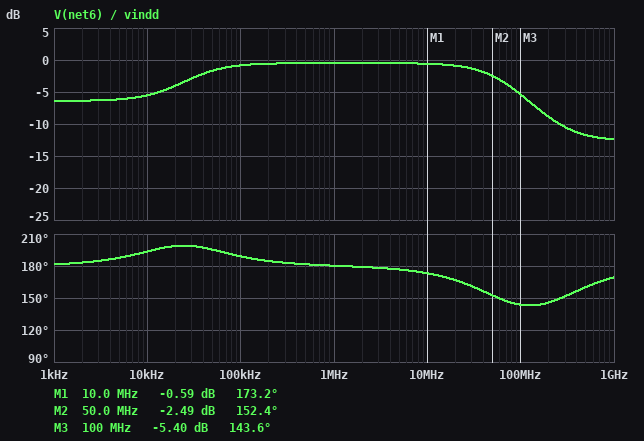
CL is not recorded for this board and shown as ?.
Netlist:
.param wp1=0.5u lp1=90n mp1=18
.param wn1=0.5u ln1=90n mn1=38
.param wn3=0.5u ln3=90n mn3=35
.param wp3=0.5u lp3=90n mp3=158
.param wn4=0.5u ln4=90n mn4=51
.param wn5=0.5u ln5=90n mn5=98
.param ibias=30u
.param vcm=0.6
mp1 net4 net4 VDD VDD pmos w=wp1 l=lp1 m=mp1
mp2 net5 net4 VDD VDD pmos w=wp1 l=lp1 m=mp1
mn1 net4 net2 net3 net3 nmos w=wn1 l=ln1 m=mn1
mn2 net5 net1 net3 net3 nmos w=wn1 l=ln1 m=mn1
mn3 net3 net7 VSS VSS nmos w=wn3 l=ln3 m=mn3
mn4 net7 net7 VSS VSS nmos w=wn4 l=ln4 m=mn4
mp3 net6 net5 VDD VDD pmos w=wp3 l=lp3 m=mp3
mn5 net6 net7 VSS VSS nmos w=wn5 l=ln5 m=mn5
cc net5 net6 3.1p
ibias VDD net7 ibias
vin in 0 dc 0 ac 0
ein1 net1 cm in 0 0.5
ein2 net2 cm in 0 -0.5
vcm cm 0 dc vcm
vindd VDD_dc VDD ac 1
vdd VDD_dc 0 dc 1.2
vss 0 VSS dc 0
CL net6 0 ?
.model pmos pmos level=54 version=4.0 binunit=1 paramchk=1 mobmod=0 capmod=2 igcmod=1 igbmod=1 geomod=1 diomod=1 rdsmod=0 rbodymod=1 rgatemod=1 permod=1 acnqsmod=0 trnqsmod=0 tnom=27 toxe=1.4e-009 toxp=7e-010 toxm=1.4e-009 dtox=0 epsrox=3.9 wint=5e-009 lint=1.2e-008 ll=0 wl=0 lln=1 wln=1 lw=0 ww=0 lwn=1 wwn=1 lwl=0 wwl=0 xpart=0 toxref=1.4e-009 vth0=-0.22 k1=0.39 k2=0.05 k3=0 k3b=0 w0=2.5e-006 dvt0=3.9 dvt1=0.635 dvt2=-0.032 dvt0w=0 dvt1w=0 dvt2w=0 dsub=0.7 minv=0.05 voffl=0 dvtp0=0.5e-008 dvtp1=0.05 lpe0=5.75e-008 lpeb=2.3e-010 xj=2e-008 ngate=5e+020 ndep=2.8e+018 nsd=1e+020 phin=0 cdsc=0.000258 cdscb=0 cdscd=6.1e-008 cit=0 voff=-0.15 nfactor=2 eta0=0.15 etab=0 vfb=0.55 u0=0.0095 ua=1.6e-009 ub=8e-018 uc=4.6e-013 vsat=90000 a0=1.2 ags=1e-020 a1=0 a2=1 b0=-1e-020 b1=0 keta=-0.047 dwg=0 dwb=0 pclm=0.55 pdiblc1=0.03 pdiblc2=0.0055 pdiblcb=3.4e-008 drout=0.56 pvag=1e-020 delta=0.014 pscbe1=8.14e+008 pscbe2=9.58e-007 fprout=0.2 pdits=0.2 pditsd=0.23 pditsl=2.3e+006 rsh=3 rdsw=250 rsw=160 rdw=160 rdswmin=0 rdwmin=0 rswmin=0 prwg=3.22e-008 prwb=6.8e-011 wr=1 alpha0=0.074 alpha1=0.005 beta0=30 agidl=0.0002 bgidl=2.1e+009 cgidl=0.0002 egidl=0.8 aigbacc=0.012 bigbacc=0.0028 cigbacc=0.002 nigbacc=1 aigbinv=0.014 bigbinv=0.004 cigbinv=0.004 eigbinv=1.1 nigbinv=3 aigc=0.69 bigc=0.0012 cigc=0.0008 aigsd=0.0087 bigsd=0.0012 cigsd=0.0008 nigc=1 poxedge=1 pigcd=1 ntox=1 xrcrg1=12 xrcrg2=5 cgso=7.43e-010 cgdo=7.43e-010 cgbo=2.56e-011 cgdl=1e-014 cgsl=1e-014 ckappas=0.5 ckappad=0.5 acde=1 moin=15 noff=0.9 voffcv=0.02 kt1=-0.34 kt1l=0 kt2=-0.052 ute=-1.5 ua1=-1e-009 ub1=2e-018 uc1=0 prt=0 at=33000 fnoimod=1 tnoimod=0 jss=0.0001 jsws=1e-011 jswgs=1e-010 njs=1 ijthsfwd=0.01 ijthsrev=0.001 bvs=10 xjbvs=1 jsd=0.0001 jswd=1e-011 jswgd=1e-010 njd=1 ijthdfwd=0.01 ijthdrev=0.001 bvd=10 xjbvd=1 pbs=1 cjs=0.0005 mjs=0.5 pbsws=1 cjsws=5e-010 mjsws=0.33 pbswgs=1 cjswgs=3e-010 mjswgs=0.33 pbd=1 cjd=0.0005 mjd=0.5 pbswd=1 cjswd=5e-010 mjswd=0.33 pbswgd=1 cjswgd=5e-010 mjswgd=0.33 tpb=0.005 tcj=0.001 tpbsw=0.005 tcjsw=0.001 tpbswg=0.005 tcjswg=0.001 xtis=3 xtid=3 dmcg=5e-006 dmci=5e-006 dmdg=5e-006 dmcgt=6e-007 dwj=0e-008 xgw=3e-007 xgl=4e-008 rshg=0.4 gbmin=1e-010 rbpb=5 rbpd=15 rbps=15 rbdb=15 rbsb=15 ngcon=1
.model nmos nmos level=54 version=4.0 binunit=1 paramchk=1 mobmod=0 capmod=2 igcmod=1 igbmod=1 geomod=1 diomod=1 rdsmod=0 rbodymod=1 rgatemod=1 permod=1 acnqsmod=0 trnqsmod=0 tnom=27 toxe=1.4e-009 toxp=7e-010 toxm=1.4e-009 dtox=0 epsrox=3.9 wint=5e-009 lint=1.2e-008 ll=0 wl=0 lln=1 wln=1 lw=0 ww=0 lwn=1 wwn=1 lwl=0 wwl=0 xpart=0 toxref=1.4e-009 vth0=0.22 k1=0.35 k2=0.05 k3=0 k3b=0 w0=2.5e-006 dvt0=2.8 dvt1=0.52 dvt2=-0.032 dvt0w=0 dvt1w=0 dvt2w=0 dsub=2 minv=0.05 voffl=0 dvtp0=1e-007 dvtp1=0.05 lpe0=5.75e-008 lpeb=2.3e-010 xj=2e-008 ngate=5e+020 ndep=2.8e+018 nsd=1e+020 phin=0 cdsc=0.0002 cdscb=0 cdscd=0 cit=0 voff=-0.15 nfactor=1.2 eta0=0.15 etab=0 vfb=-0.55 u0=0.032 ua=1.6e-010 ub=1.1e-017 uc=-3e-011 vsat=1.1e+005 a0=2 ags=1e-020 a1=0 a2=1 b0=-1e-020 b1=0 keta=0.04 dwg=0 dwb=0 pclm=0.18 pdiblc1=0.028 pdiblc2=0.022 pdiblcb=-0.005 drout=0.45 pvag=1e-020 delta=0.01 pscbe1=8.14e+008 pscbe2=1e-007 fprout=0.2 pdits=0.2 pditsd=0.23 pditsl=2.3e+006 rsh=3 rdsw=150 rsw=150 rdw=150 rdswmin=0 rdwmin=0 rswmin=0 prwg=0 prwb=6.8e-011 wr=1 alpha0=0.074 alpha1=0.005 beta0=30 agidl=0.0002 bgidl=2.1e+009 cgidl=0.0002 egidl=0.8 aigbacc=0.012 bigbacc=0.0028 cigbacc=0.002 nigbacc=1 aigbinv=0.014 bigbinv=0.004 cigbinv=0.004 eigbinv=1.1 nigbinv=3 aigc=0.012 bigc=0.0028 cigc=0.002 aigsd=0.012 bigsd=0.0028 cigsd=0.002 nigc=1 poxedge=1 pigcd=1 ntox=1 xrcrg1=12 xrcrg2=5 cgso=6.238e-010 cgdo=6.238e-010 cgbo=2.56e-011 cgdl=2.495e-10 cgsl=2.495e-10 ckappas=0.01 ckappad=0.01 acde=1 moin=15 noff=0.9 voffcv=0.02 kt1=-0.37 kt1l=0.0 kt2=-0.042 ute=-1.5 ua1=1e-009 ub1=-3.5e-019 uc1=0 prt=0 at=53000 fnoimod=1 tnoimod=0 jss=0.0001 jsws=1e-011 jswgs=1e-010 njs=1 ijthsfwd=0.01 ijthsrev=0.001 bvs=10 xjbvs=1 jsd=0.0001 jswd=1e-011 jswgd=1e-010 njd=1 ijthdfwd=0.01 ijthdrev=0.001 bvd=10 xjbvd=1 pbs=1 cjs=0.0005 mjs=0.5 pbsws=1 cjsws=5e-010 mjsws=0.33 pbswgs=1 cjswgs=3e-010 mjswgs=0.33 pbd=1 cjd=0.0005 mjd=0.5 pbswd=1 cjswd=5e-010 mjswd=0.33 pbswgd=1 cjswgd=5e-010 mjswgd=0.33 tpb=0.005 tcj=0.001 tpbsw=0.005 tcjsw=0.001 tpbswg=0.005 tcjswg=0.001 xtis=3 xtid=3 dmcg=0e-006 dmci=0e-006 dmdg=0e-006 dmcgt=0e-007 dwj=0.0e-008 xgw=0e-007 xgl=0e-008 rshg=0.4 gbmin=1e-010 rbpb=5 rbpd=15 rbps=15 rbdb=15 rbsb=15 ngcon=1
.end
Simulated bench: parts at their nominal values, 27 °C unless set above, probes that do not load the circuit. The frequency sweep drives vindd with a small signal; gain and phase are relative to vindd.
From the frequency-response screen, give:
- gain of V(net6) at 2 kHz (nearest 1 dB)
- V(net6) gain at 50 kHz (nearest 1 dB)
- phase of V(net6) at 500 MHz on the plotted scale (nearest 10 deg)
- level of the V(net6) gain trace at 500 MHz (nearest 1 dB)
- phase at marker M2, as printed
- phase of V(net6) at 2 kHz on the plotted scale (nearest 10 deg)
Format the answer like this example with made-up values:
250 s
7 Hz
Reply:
-6 dB
-2 dB
160 deg
-12 dB
152.4 deg
180 deg
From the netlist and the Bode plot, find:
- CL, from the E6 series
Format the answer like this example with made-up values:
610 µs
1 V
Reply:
3.3 pF
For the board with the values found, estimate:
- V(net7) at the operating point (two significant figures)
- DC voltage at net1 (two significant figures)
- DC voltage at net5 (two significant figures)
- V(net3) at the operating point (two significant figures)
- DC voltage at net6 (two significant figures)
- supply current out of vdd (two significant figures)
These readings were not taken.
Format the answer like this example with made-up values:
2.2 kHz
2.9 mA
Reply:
300 mV
600 mV
870 mV
340 mV
940 mV
140 µA
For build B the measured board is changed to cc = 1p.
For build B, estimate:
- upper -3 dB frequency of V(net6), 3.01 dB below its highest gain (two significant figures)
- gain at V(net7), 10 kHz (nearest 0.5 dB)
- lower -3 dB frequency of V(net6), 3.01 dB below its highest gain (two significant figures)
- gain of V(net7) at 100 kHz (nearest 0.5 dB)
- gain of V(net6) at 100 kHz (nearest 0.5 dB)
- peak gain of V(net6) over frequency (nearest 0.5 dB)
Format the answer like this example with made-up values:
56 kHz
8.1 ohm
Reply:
60 MHz
-43.5 dB
68 kHz
-39.5 dB
-2.5 dB
-0.5 dB
